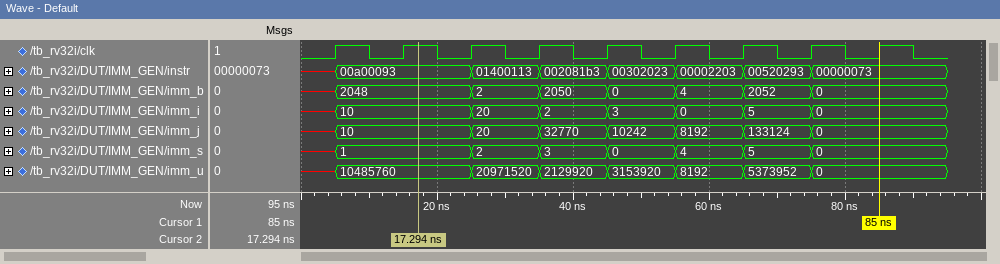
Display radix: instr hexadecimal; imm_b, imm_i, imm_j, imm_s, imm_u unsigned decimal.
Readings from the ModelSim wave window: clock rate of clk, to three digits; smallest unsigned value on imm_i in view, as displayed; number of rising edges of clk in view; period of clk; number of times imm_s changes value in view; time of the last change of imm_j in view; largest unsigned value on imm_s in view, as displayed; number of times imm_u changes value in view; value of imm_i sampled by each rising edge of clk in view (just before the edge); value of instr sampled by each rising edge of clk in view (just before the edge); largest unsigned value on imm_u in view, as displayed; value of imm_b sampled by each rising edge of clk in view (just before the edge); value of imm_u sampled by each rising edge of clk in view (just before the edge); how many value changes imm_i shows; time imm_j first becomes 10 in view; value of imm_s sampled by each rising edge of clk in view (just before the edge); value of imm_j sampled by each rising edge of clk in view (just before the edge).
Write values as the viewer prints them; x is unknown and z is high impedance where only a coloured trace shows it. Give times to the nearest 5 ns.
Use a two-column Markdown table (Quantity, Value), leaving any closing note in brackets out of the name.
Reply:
| Quantity | Value |
|---|---|
| clock rate of clk, to three digits | 100 MHz |
| smallest unsigned value on imm_i in view, as displayed | 0 |
| number of rising edges of clk in view | 9 |
| period of clk | 10 ns |
| number of times imm_s changes value in view | 7 |
| time of the last change of imm_j in view | 75 ns |
| largest unsigned value on imm_s in view, as displayed | 5 |
| number of times imm_u changes value in view | 7 |
| value of imm_i sampled by each rising edge of clk in view | x, 10, 10, 20, 2, 3, 0, 5, 0 |
| value of instr sampled by each rising edge of clk in view | x, 00a00093, 00a00093, 01400113, 002081b3, 00302023, 00002203, 00520293, 00000073 |
| largest unsigned value on imm_u in view, as displayed | 20971520 |
| value of imm_b sampled by each rising edge of clk in view | x, 2048, 2048, 2, 2050, 0, 4, 2052, 0 |
| value of imm_u sampled by each rising edge of clk in view | x, 10485760, 10485760, 20971520, 2129920, 3153920, 8192, 5373952, 0 |
| how many value changes imm_i shows | 7 |
| time imm_j first becomes 10 in view | 5 ns |
| value of imm_s sampled by each rising edge of clk in view | x, 1, 1, 2, 3, 0, 4, 5, 0 |
| value of imm_j sampled by each rising edge of clk in view | x, 10, 10, 20, 32770, 10242, 8192, 133124, 0 |
